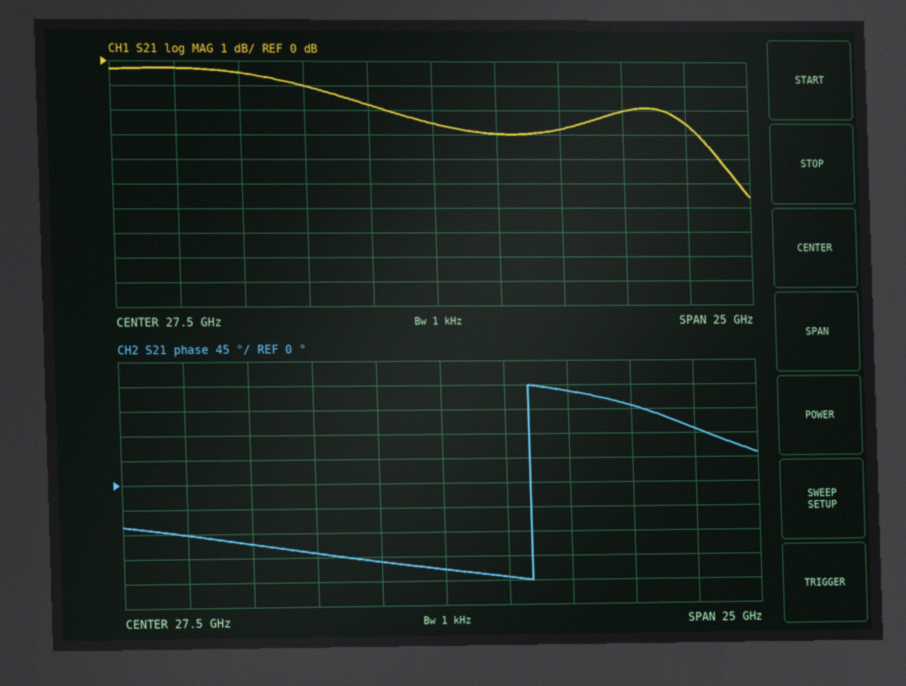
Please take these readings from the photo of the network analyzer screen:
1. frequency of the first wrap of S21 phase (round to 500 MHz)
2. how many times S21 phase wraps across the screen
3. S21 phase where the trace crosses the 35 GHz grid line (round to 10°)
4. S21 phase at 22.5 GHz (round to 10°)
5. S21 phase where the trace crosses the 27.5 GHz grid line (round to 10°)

31.0 GHz
1
140°
-130°
-160°
